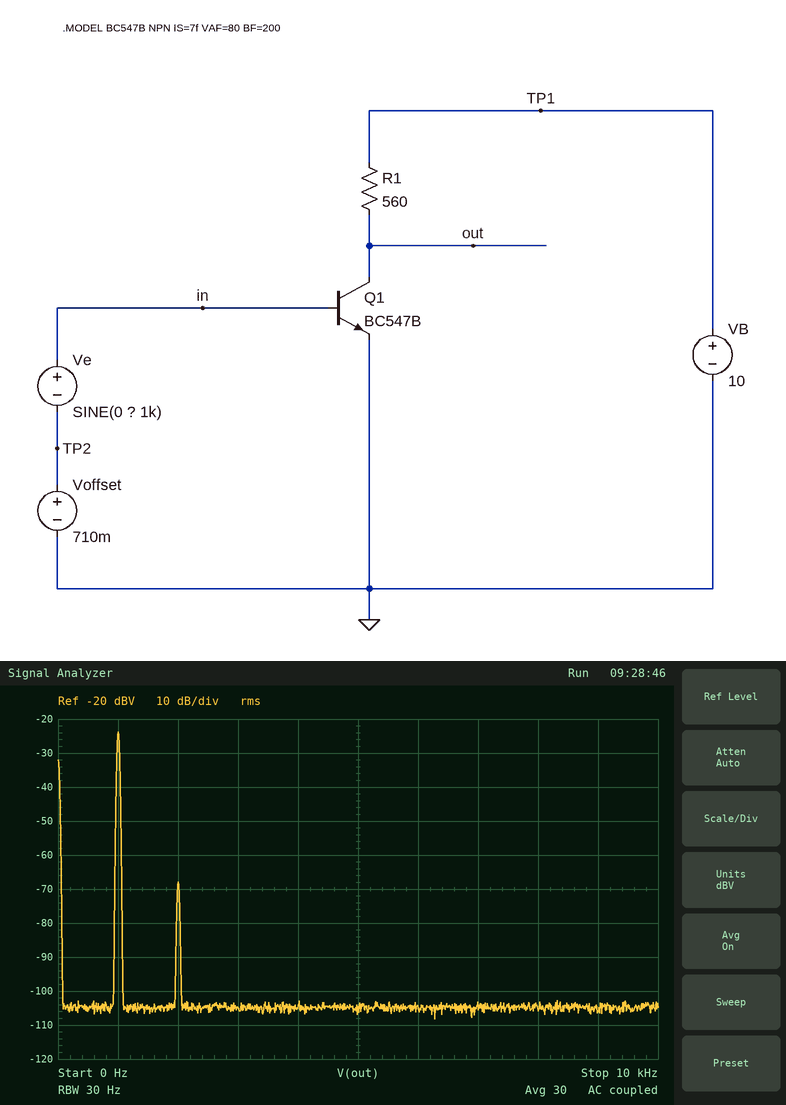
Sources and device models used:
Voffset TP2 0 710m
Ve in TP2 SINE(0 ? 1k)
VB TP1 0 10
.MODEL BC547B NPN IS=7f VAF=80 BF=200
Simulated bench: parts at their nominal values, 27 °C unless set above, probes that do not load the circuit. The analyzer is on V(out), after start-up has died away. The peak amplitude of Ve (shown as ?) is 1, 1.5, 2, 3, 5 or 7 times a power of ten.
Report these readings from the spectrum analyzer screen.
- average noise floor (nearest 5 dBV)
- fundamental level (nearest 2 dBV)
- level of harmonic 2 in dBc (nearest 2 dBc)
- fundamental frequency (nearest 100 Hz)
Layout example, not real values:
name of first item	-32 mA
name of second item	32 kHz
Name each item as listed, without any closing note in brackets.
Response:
average noise floor	-105 dBV
fundamental level	-24 dBV
level of harmonic 2 in dBc	-44 dBc
fundamental frequency	1.0 kHz
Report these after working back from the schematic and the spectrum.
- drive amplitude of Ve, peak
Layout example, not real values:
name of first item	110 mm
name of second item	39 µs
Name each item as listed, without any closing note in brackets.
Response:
drive amplitude of Ve, peak	700 µV
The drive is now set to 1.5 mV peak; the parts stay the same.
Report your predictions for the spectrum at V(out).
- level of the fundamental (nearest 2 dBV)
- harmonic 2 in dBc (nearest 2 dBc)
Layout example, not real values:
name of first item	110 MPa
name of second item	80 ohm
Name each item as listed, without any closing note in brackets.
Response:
level of the fundamental	-18 dBV
harmonic 2 in dBc	-38 dBc
